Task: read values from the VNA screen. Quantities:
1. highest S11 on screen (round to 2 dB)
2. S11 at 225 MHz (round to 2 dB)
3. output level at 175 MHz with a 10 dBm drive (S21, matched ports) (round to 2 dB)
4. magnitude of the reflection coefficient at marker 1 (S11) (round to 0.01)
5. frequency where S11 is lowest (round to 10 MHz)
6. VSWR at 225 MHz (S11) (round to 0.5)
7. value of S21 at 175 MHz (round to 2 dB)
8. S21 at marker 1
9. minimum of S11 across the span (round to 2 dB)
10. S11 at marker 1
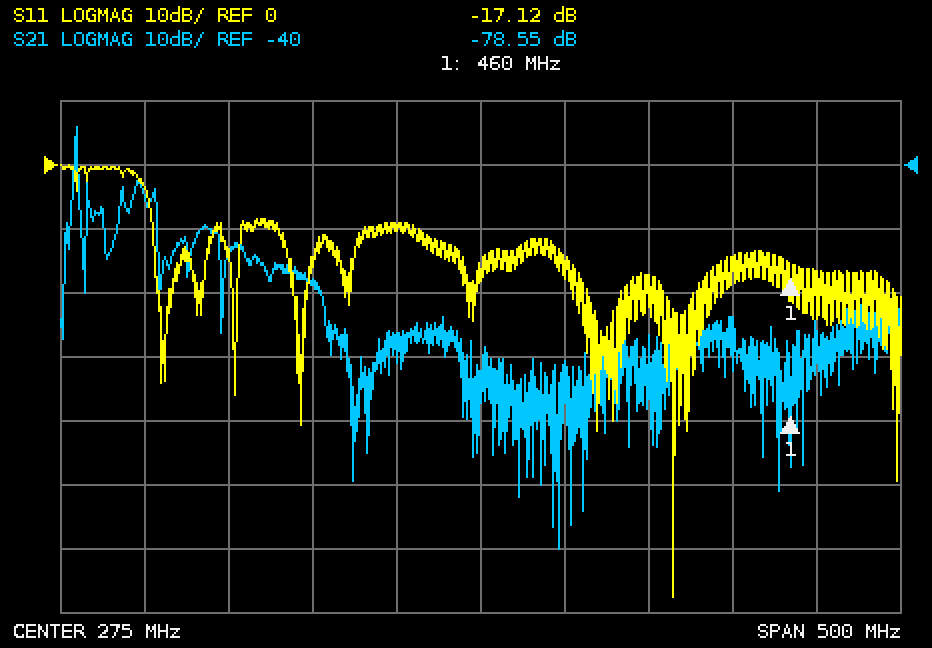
0 dB
-10 dB
-48 dBm
0.14
390 MHz
2.0
-58 dB
-78.55 dB
-68 dB
-17.12 dB
